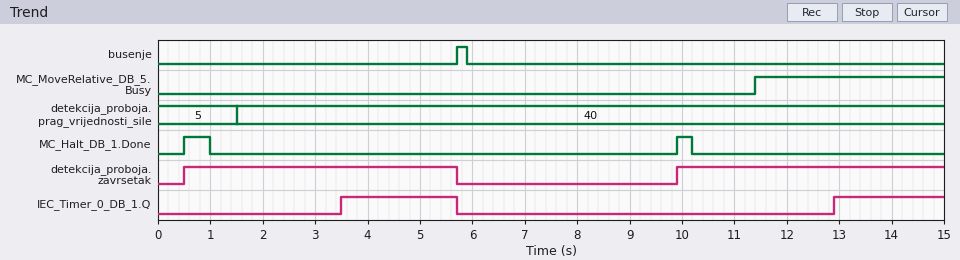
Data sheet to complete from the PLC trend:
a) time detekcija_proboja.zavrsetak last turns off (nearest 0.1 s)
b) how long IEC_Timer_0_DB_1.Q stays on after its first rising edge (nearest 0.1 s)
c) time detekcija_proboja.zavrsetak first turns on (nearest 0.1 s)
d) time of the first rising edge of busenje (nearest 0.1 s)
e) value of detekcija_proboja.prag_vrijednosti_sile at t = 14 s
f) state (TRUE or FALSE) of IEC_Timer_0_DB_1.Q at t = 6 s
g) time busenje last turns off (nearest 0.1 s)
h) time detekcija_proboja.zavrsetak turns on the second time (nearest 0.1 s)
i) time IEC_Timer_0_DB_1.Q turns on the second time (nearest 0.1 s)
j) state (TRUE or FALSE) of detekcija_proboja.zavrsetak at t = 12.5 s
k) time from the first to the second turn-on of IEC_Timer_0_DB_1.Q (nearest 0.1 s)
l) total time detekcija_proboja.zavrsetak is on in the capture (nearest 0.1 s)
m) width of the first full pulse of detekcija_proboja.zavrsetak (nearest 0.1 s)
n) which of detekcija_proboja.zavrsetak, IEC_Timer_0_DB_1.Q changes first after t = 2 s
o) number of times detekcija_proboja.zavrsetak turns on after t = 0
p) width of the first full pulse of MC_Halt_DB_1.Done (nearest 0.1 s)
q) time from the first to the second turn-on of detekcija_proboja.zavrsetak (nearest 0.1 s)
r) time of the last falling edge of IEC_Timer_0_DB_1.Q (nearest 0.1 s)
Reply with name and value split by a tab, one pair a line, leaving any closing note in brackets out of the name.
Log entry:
time detekcija_proboja.zavrsetak last turns off	5.7 s
how long IEC_Timer_0_DB_1.Q stays on after its first rising edge	2.2 s
time detekcija_proboja.zavrsetak first turns on	0.5 s
time of the first rising edge of busenje	5.7 s
value of detekcija_proboja.prag_vrijednosti_sile at t = 14 s	40
state (TRUE or FALSE) of IEC_Timer_0_DB_1.Q at t = 6 s	FALSE
time busenje last turns off	5.9 s
time detekcija_proboja.zavrsetak turns on the second time	9.9 s
time IEC_Timer_0_DB_1.Q turns on the second time	12.9 s
state (TRUE or FALSE) of detekcija_proboja.zavrsetak at t = 12.5 s	TRUE
time from the first to the second turn-on of IEC_Timer_0_DB_1.Q	9.4 s
total time detekcija_proboja.zavrsetak is on in the capture	10.3 s
width of the first full pulse of detekcija_proboja.zavrsetak	5.2 s
which of detekcija_proboja.zavrsetak, IEC_Timer_0_DB_1.Q changes first after t = 2 s	IEC_Timer_0_DB_1.Q
number of times detekcija_proboja.zavrsetak turns on after t = 0	2
width of the first full pulse of MC_Halt_DB_1.Done	0.5 s
time from the first to the second turn-on of detekcija_proboja.zavrsetak	9.4 s
time of the last falling edge of IEC_Timer_0_DB_1.Q	5.7 s
